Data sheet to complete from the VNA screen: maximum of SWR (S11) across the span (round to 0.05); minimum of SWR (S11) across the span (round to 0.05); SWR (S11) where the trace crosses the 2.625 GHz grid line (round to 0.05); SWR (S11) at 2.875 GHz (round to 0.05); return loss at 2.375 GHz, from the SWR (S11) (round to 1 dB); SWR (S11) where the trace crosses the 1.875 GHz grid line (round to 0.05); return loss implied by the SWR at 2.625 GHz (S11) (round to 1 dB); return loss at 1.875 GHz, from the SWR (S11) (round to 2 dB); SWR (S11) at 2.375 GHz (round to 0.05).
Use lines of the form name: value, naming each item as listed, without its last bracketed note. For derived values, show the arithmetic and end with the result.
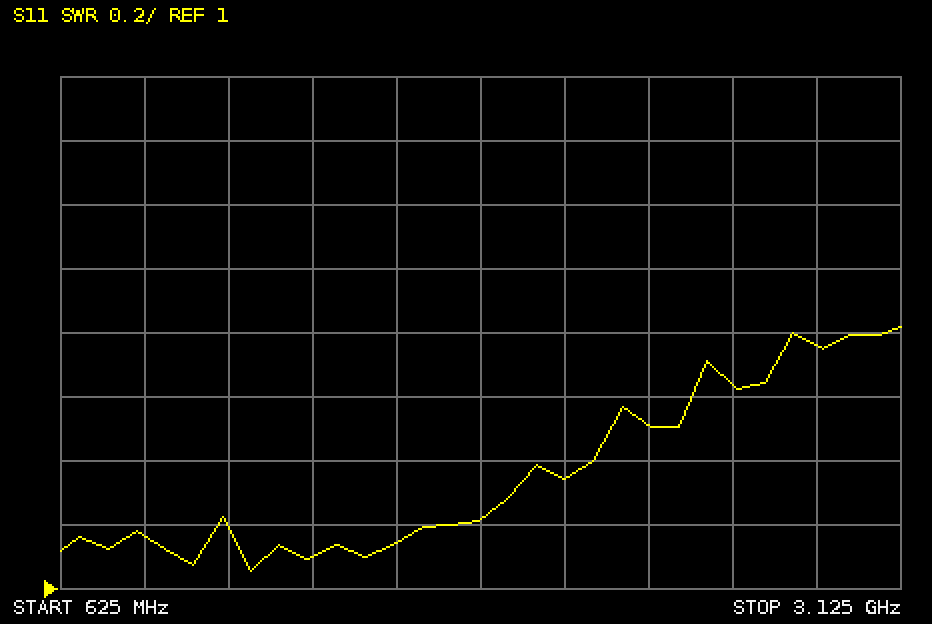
maximum of SWR (S11) across the span: 1.80
minimum of SWR (S11) across the span: 1.05
SWR (S11) where the trace crosses the 2.625 GHz grid line: 1.65
SWR (S11) at 2.875 GHz: 1.75
return loss at 2.375 GHz, from the SWR (S11): −20 log10((1.5 − 1)/(1.5 + 1)) ≈ 14 dB
SWR (S11) where the trace crosses the 1.875 GHz grid line: 1.20
return loss implied by the SWR at 2.625 GHz (S11): −20 log10((1.65 − 1)/(1.65 + 1)) ≈ 12 dB
return loss at 1.875 GHz, from the SWR (S11): −20 log10((1.2 − 1)/(1.2 + 1)) ≈ 20.8 dB, so 20 dB to the nearest 2 dB
SWR (S11) at 2.375 GHz: 1.50
